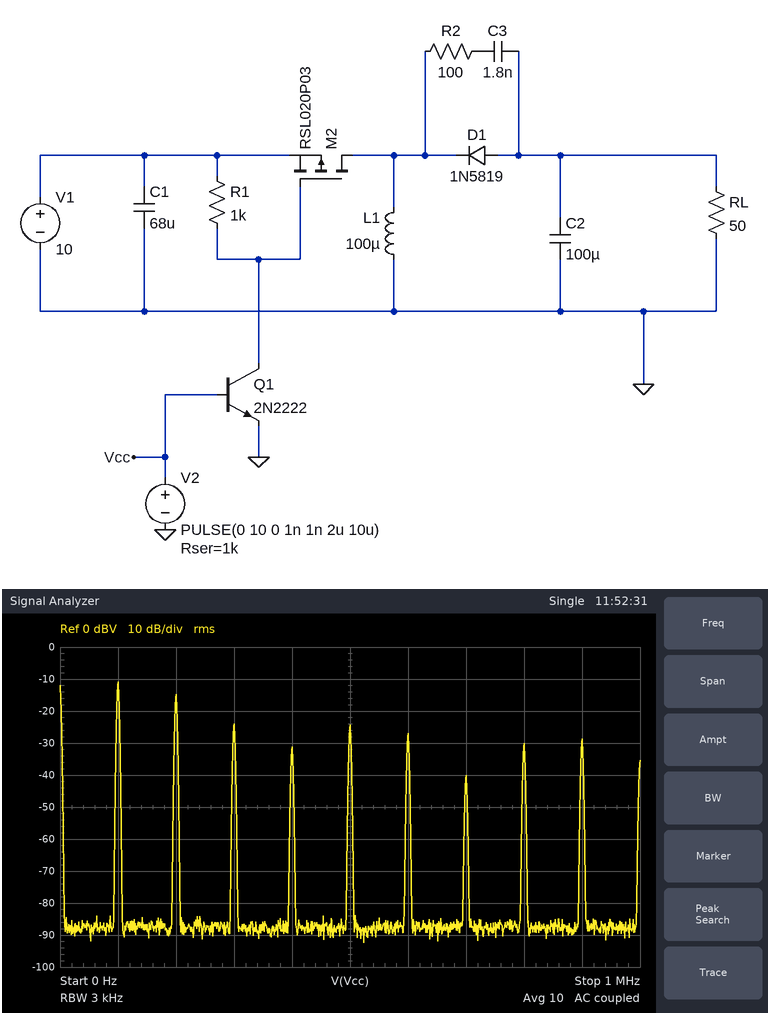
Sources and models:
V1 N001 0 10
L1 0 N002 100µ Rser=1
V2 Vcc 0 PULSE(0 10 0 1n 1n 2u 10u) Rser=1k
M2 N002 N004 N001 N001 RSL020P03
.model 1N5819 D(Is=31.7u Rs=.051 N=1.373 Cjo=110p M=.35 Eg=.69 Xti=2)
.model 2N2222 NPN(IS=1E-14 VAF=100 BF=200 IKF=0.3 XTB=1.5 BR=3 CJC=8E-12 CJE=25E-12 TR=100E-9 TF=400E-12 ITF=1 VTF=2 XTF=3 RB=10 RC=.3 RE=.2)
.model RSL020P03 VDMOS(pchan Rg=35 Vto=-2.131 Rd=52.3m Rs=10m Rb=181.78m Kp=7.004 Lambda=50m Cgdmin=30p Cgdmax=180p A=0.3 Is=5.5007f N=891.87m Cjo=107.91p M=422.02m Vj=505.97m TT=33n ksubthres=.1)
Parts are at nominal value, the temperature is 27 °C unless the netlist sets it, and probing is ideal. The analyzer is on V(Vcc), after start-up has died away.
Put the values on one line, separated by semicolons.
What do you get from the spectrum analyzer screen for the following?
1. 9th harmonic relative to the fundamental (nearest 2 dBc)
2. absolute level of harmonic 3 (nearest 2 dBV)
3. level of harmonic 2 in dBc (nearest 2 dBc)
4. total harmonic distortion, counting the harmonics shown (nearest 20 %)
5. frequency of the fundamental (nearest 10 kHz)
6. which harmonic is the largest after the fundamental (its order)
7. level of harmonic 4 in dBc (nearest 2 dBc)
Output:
-18 dBc; -24 dBV; -4 dBc; 80 %; 100 kHz; 2; -20 dBc
